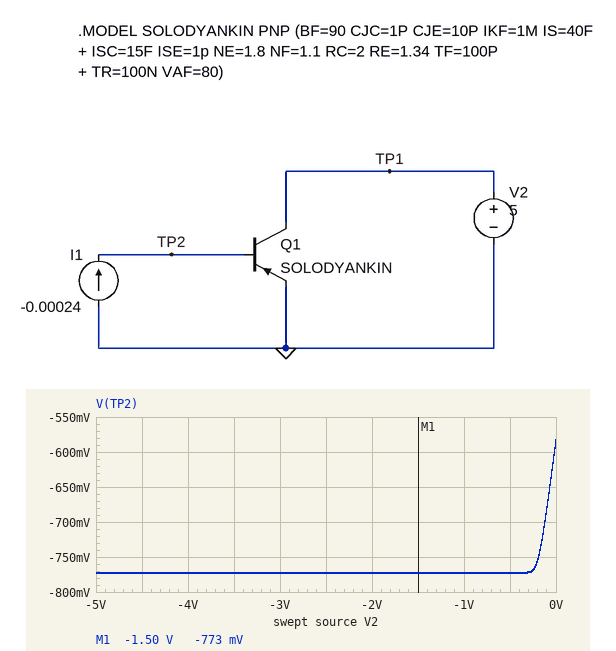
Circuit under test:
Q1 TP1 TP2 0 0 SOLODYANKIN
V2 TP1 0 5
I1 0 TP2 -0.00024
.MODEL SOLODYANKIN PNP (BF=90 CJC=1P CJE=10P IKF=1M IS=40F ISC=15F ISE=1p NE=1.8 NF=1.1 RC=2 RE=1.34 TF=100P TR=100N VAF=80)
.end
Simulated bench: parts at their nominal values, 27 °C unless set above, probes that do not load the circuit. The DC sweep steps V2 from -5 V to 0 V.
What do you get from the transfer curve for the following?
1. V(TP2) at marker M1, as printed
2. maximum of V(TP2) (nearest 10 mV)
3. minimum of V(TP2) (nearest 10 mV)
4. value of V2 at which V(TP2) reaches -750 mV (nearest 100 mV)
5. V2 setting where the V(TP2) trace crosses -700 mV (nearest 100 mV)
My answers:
-773 mV
-580 mV
-770 mV
-200 mV
-100 mV
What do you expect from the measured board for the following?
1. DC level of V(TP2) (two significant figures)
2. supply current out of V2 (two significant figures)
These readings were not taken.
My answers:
4.4 V
480 µA
